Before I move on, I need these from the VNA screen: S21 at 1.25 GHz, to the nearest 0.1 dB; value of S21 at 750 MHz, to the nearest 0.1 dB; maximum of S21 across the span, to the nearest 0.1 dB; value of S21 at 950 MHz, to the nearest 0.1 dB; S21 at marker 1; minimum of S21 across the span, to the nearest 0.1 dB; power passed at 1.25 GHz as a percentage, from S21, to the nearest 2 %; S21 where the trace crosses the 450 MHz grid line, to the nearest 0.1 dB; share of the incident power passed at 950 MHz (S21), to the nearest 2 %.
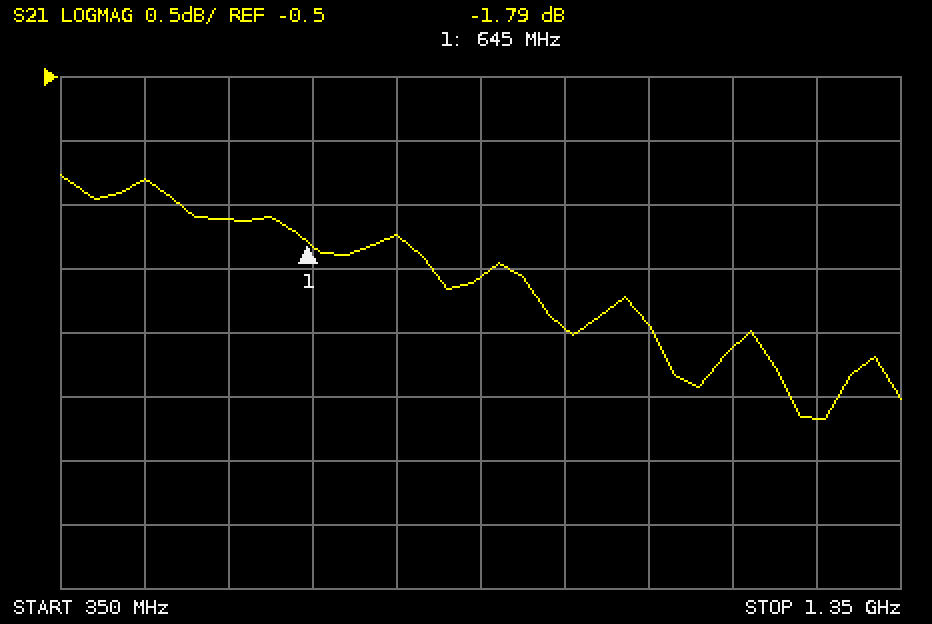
-3.2 dB
-1.7 dB
-1.3 dB
-2.5 dB
-1.79 dB
-3.2 dB
48 %
-1.3 dB
56 %
